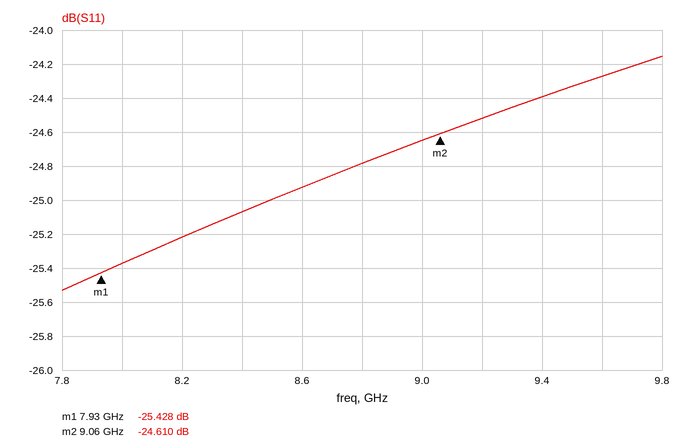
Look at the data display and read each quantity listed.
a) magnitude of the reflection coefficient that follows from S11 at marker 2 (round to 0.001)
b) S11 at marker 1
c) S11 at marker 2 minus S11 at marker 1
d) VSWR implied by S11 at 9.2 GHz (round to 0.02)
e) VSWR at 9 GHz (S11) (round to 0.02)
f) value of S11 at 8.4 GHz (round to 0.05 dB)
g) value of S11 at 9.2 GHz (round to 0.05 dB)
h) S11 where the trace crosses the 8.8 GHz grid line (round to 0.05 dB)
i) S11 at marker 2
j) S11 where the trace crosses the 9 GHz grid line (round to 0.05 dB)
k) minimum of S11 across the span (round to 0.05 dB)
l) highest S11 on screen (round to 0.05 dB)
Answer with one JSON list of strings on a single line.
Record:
["0.059", "-25.428 dB", "0.818 dB", "1.12", "1.12", "-25.05 dB", "-24.50 dB", "-24.80 dB", "-24.610 dB", "-24.65 dB", "-25.55 dB", "-24.15 dB"]
